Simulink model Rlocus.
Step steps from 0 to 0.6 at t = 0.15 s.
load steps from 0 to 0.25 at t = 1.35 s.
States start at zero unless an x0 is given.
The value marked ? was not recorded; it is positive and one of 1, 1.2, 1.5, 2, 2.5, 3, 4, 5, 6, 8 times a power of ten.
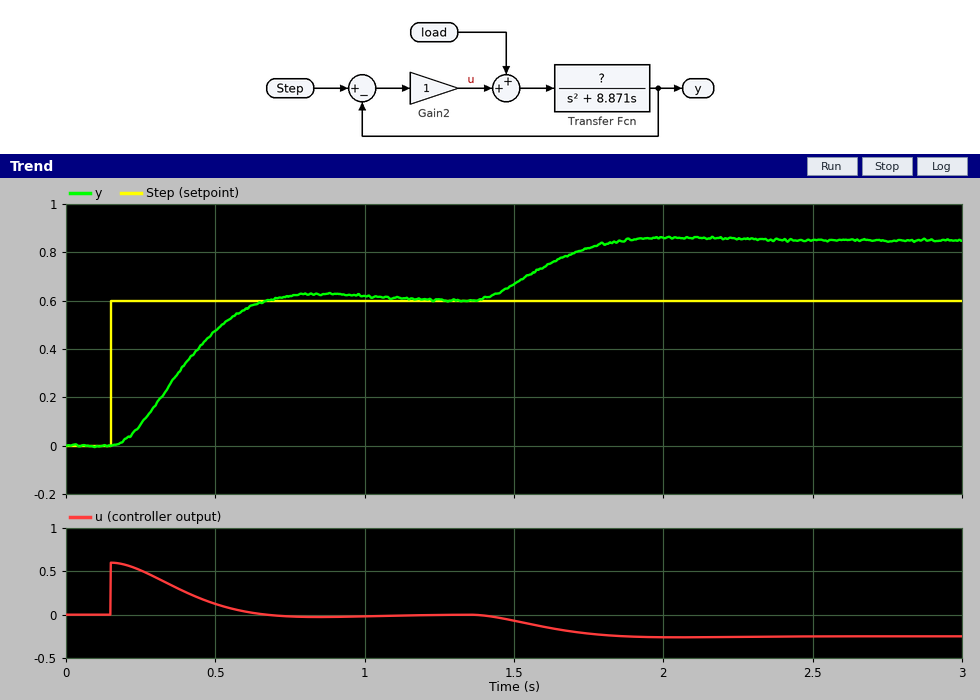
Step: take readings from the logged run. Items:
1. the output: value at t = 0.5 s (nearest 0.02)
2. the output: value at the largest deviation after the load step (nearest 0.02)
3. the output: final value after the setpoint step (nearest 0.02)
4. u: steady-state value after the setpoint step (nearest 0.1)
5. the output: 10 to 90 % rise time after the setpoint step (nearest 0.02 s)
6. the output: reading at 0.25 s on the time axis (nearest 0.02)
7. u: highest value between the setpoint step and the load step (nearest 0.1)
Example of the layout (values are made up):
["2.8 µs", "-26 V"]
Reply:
["0.48", "0.86", "0.60", "0.0", "0.34 s", "0.08", "0.6"]
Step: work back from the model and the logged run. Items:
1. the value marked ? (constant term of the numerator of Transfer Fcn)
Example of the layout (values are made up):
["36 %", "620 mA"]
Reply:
["40"]
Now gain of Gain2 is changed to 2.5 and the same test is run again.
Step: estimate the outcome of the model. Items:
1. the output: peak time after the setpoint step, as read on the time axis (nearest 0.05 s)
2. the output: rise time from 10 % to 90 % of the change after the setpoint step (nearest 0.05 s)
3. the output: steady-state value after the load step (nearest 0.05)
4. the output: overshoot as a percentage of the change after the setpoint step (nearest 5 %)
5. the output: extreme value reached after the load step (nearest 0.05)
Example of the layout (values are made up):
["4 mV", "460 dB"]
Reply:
["0.50 s", "0.15 s", "0.70", "20 %", "0.70"]
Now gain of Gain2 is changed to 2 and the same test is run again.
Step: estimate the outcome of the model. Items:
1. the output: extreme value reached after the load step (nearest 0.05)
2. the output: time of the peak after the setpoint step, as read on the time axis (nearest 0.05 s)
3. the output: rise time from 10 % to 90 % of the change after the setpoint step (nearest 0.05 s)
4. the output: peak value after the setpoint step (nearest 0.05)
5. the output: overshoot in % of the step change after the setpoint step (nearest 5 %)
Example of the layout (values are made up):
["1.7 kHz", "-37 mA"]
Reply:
["0.75", "0.55 s", "0.20 s", "0.70", "15 %"]
